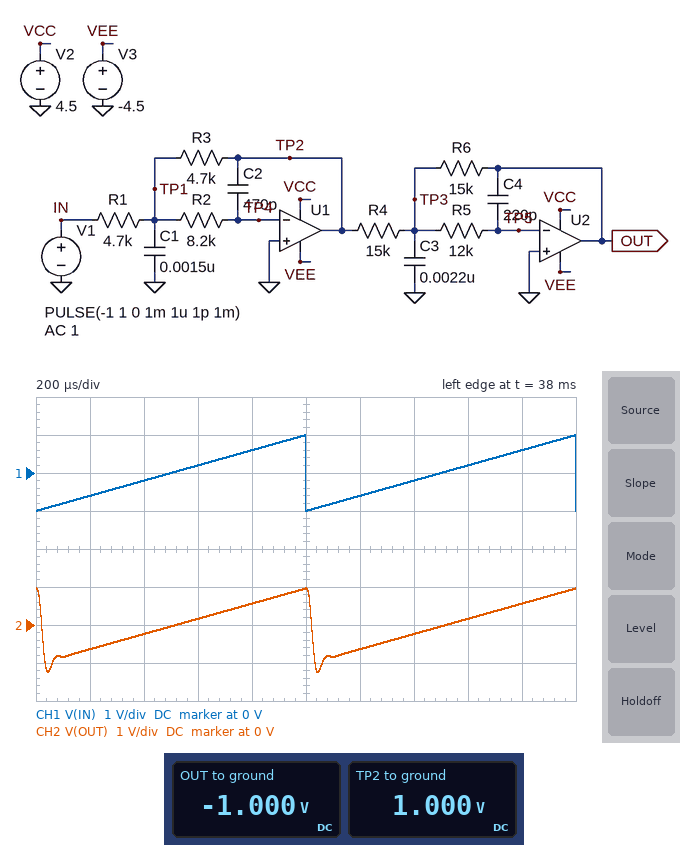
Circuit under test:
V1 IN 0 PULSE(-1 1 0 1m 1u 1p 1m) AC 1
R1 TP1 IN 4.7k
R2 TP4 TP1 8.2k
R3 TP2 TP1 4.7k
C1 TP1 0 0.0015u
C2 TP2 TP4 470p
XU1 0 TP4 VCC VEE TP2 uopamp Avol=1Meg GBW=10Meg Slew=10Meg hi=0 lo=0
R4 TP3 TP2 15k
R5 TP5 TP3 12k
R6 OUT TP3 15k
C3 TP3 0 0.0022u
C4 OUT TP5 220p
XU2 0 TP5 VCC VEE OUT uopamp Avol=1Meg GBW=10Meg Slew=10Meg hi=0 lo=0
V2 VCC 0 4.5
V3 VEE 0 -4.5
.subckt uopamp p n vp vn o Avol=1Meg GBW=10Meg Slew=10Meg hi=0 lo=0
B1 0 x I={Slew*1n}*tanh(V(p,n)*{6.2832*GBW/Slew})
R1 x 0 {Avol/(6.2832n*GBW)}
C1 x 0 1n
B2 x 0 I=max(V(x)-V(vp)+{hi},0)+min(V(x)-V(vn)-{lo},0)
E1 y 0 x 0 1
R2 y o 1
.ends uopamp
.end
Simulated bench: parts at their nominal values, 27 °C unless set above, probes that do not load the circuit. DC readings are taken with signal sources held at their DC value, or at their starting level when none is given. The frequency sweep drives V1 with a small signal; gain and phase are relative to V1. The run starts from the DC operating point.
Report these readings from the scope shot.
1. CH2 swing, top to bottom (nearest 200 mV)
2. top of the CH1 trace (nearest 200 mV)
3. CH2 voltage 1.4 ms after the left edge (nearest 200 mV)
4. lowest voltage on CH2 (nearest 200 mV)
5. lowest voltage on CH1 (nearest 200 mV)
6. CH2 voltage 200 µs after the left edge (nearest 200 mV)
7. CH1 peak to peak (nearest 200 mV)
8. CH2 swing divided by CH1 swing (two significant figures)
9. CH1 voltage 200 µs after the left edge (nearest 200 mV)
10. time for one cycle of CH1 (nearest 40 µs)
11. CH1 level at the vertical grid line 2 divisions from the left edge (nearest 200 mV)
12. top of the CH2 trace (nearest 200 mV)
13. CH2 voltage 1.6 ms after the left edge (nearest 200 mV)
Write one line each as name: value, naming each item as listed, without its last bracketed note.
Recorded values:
CH2 swing, top to bottom: 2.2 V
top of the CH1 trace: 1.0 V
CH2 voltage 1.4 ms after the left edge: -200 mV
lowest voltage on CH2: -1.2 V
lowest voltage on CH1: -1.0 V
CH2 voltage 200 µs after the left edge: -600 mV
CH1 peak to peak: 2.0 V
CH2 swing divided by CH1 swing: 1.1
CH1 voltage 200 µs after the left edge: -600 mV
time for one cycle of CH1: 1.00 ms
CH1 level at the vertical grid line 2 divisions from the left edge: -200 mV
top of the CH2 trace: 1.0 V
CH2 voltage 1.6 ms after the left edge: 200 mV
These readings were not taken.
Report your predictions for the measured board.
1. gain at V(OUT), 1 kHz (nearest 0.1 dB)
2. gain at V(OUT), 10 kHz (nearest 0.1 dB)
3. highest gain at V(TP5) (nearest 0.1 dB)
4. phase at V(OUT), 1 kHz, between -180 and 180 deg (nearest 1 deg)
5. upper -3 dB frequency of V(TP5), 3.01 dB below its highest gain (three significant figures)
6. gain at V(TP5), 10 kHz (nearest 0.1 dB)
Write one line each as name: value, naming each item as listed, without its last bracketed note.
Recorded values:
gain at V(OUT), 1 kHz: 0 dB
gain at V(OUT), 10 kHz: 0.7 dB
highest gain at V(TP5): -56.5 dB
phase at V(OUT), 1 kHz, between -180 and 180 deg: -7 deg
upper -3 dB frequency of V(TP5), 3.01 dB below its highest gain: 22.7 kHz
gain at V(TP5), 10 kHz: -59.3 dB
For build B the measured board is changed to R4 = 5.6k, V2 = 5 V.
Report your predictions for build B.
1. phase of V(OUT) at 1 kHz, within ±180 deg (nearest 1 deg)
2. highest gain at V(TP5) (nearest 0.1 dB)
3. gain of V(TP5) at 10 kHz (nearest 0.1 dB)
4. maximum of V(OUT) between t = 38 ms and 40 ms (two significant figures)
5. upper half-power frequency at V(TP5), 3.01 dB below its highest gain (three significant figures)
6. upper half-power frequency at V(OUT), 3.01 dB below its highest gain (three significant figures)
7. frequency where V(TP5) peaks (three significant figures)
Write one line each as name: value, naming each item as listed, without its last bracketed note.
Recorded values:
phase of V(OUT) at 1 kHz, within ±180 deg: -8 deg
highest gain at V(TP5): -51.5 dB
gain of V(TP5) at 10 kHz: -52.6 dB
maximum of V(OUT) between t = 38 ms and 40 ms: 2.6 V
upper half-power frequency at V(TP5), 3.01 dB below its highest gain: 24.0 kHz
upper half-power frequency at V(OUT), 3.01 dB below its highest gain: 14.1 kHz
frequency where V(TP5) peaks: 14.4 kHz
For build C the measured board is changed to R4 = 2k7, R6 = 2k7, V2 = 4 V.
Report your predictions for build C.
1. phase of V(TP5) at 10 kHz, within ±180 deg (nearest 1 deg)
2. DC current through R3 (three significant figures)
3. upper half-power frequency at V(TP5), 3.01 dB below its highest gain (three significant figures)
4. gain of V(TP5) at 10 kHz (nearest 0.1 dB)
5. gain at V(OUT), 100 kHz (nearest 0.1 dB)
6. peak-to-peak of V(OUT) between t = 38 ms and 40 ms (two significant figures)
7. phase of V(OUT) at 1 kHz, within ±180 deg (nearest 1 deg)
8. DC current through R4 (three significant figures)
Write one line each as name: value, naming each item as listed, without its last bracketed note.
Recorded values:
phase of V(TP5) at 10 kHz, within ±180 deg: -147 deg
DC current through R3: 213 µA
upper half-power frequency at V(TP5), 3.01 dB below its highest gain: 41.1 kHz
gain of V(TP5) at 10 kHz: -60.8 dB
gain at V(OUT), 100 kHz: -37.4 dB
peak-to-peak of V(OUT) between t = 38 ms and 40 ms: 1.9 V
phase of V(OUT) at 1 kHz, within ±180 deg: -6 deg
DC current through R4: 370 µA
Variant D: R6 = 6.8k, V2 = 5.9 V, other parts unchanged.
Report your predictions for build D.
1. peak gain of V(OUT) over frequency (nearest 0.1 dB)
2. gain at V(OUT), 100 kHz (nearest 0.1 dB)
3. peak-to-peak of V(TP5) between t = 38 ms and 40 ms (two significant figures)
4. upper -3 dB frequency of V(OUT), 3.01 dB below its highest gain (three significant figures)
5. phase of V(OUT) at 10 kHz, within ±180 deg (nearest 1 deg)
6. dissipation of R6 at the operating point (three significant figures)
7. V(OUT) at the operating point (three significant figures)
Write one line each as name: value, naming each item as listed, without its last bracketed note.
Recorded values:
peak gain of V(OUT) over frequency: -6.7 dB
gain at V(OUT), 100 kHz: -51.7 dB
peak-to-peak of V(TP5) between t = 38 ms and 40 ms: 1.1 mV
upper -3 dB frequency of V(OUT), 3.01 dB below its highest gain: 25.6 kHz
phase of V(OUT) at 10 kHz, within ±180 deg: -57 deg
dissipation of R6 at the operating point: 30.2 µW
V(OUT) at the operating point: -453 mV
